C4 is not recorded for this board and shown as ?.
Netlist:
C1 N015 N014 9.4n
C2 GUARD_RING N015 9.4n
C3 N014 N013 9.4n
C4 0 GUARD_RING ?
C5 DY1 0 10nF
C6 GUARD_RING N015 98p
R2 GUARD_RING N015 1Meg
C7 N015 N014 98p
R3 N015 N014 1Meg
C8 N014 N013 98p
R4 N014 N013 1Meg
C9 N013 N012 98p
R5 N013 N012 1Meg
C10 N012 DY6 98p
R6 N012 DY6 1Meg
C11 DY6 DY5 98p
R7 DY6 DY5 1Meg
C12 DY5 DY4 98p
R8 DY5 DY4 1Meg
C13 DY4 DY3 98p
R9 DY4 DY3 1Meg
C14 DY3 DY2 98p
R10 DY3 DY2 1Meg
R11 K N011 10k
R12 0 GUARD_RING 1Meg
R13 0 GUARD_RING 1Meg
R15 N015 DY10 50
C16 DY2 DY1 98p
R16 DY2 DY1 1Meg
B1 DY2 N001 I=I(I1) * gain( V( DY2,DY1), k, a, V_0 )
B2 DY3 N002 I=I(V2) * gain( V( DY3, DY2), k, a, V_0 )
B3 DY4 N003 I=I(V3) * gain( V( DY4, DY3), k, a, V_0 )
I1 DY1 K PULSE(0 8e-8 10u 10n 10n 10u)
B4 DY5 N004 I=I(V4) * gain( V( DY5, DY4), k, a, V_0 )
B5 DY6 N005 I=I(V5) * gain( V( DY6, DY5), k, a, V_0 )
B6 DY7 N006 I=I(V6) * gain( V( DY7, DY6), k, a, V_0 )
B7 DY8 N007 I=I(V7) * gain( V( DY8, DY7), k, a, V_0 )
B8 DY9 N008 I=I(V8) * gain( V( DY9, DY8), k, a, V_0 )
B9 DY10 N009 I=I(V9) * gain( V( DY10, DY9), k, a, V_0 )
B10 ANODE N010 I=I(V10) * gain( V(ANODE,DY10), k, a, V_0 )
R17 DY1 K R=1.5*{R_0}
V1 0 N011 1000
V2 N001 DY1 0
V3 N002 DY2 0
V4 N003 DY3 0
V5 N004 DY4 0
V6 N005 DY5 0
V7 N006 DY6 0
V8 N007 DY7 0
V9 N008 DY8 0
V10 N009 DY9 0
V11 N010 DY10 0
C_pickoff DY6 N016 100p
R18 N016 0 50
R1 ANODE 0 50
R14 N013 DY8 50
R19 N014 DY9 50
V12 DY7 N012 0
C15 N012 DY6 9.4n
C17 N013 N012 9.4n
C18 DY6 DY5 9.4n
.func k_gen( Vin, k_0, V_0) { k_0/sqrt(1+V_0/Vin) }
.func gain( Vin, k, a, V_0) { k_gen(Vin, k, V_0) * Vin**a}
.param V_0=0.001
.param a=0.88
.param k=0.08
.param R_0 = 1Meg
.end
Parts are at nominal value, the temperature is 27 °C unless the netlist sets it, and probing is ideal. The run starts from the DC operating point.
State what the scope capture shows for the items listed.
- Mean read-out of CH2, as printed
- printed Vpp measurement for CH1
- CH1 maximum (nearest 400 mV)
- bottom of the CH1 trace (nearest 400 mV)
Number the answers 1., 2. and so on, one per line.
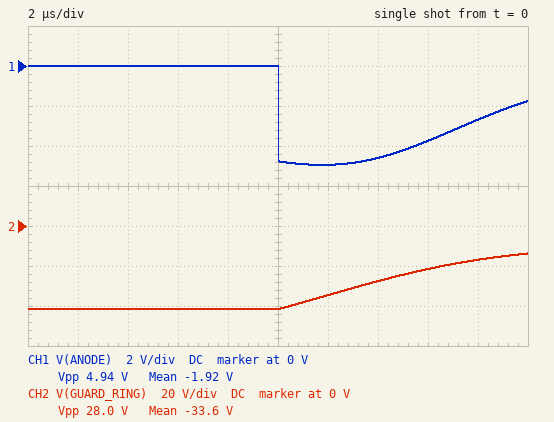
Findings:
1. -33.6 V
2. 4.94 V
3. 0 V
4. -4.8 V
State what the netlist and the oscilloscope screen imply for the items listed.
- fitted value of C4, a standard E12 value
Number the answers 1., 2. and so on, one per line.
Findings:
1. 27 nF
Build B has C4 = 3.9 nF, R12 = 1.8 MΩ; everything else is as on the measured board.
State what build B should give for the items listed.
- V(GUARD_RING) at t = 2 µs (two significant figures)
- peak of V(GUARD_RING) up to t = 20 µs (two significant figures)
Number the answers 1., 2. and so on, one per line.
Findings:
1. -53 V
2. 44 V
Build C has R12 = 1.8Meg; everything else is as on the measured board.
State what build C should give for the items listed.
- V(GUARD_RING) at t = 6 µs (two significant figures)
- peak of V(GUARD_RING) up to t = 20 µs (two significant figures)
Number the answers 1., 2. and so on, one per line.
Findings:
1. -53 V
2. -23 V
